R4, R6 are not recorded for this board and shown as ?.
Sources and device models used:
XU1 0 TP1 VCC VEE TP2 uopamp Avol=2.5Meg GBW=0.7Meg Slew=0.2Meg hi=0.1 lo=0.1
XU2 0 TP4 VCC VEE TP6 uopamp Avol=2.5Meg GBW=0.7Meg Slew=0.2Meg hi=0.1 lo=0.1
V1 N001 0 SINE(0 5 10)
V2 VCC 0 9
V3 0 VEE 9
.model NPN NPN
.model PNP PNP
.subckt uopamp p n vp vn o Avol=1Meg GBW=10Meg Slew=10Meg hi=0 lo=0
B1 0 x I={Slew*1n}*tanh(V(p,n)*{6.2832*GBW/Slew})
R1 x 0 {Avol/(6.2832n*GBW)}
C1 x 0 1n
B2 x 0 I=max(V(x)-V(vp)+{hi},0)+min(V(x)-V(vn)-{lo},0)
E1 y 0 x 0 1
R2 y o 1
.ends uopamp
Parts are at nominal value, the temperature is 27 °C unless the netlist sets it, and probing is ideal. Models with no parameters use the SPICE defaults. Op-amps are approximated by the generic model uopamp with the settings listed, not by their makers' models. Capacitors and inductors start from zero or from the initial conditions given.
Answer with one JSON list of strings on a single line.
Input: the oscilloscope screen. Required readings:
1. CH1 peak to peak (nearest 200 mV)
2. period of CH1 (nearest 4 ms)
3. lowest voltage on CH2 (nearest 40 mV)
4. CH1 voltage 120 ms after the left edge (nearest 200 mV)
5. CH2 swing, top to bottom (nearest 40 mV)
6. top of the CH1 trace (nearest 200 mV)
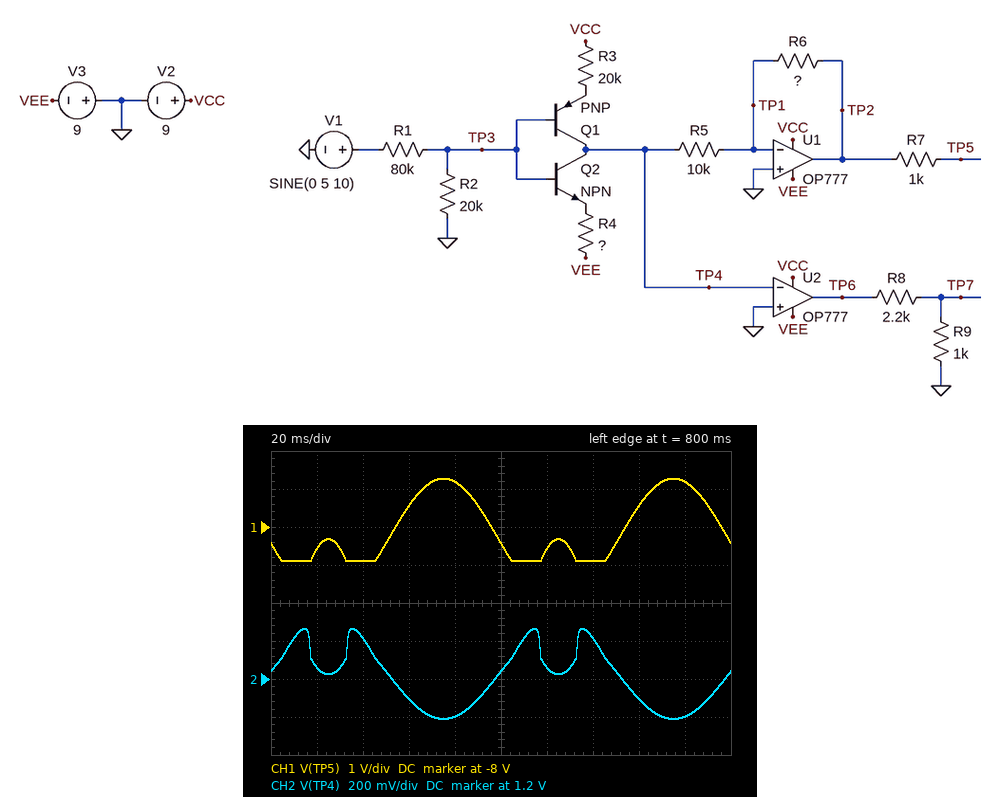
["2.2 V", "100 ms", "1.00 V", "-8.6 V", "480 mV", "-6.8 V"]
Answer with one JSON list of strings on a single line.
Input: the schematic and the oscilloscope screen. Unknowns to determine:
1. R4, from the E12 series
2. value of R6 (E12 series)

["39 kΩ", "68 kΩ"]
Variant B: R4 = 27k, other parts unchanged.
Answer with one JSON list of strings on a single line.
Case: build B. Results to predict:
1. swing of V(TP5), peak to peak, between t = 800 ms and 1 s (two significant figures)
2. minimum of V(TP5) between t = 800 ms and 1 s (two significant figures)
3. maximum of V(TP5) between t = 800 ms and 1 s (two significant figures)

["3.7 V", "-5.7 V", "-2.0 V"]
